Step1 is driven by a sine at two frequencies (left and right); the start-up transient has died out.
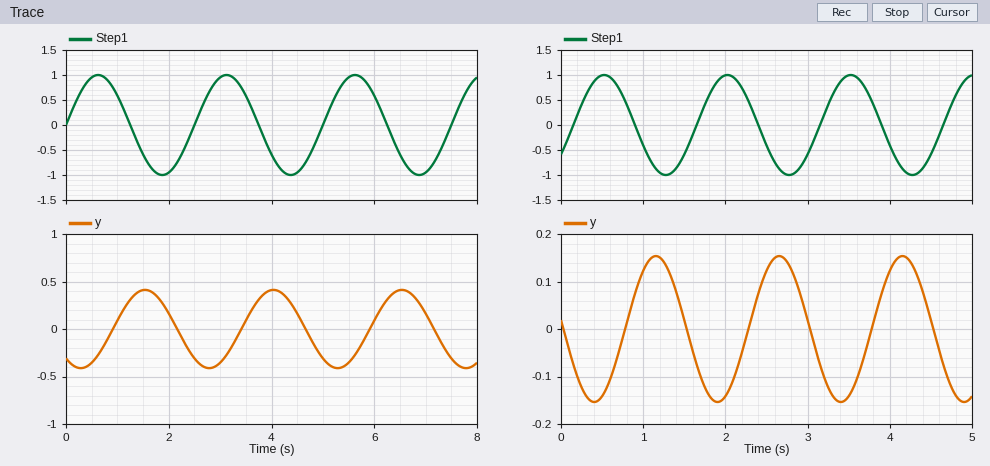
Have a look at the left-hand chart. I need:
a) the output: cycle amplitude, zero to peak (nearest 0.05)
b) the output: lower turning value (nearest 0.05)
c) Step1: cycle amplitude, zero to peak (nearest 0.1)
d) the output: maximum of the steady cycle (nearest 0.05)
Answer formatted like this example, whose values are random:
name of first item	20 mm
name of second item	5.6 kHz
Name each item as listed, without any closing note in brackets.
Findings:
the output: cycle amplitude, zero to peak	0.40
the output: lower turning value	-0.40
Step1: cycle amplitude, zero to peak	1.0
the output: maximum of the steady cycle	0.40
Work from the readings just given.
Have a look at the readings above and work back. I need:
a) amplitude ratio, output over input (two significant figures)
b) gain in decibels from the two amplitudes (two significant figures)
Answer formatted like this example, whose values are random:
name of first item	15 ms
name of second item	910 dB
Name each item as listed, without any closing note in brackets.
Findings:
amplitude ratio, output over input	0.40
gain in decibels from the two amplitudes	-8.0 dB
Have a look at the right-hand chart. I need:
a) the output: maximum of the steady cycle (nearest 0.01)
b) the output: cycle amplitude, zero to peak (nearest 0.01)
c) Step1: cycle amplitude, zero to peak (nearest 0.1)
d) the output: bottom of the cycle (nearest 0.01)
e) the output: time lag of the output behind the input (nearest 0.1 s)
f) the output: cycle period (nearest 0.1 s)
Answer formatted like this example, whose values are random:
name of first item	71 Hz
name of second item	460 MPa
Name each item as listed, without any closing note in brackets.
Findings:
the output: maximum of the steady cycle	0.15
the output: cycle amplitude, zero to peak	0.15
Step1: cycle amplitude, zero to peak	1.0
the output: bottom of the cycle	-0.15
the output: time lag of the output behind the input	0.6 s
the output: cycle period	1.5 s
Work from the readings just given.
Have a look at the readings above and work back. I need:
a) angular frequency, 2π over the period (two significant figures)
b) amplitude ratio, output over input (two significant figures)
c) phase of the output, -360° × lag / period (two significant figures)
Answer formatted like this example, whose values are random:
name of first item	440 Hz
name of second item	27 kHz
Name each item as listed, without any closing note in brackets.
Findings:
angular frequency, 2π over the period	4.2 rad/s
amplitude ratio, output over input	0.15
phase of the output, -360° × lag / period	-140°
